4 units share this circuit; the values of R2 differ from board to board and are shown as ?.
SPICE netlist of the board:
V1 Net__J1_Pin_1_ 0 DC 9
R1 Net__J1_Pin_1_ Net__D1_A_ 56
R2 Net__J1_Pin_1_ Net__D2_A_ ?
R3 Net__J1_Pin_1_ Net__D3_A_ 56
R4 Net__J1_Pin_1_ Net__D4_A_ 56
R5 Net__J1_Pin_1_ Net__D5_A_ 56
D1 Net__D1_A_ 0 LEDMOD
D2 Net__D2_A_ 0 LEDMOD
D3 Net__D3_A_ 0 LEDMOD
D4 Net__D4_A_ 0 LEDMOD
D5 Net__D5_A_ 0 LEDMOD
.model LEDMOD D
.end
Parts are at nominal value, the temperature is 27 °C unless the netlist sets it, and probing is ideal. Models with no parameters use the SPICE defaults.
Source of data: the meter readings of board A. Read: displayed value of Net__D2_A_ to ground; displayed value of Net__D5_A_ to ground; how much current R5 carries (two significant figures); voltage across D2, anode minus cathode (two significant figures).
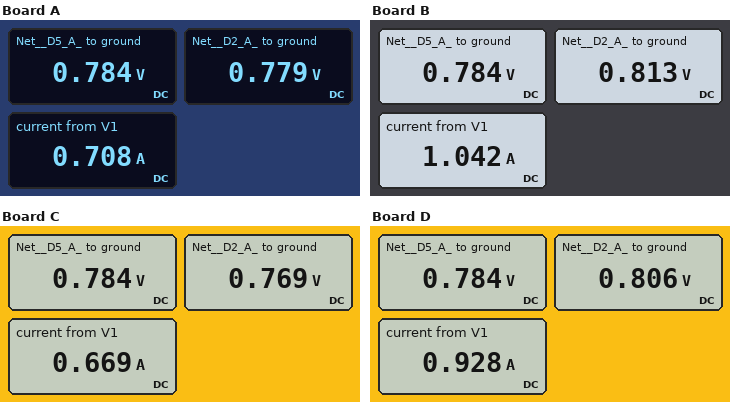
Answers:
0.779 V
0.784 V
150 mA
780 mV
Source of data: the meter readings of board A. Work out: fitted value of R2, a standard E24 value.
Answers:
68 Ω
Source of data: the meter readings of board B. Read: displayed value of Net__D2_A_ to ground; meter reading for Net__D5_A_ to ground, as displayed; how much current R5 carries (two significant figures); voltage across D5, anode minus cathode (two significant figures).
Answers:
0.813 V
0.784 V
150 mA
780 mV
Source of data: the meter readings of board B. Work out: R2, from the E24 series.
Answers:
18 Ω
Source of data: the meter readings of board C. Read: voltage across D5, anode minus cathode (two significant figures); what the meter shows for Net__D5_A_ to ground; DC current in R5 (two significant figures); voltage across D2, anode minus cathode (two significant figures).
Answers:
780 mV
0.784 V
150 mA
770 mV
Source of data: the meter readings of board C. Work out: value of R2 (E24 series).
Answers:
100 Ω
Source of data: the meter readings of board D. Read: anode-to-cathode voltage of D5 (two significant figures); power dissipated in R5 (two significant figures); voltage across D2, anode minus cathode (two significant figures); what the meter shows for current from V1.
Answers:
780 mV
1.2 W
810 mV
0.928 A
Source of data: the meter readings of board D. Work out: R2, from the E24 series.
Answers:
24 Ω
